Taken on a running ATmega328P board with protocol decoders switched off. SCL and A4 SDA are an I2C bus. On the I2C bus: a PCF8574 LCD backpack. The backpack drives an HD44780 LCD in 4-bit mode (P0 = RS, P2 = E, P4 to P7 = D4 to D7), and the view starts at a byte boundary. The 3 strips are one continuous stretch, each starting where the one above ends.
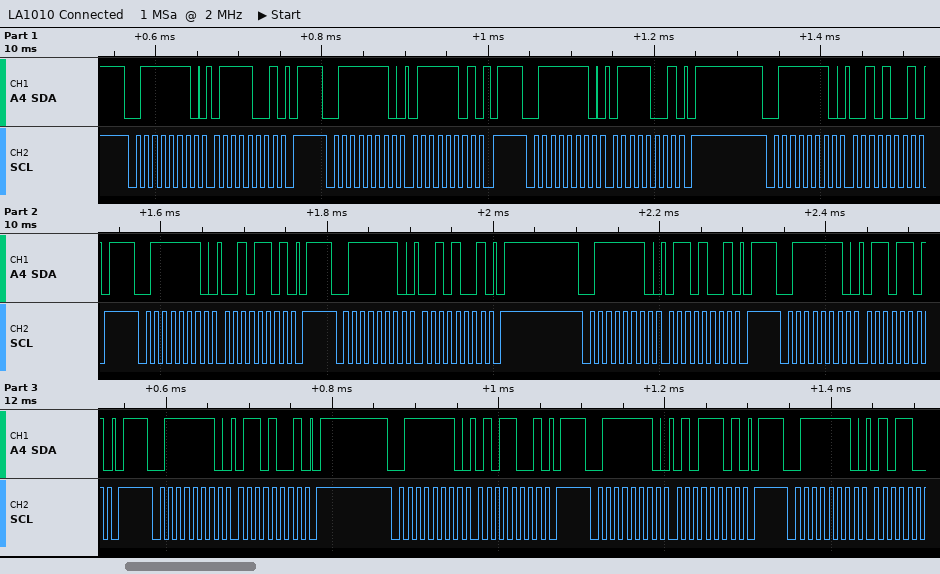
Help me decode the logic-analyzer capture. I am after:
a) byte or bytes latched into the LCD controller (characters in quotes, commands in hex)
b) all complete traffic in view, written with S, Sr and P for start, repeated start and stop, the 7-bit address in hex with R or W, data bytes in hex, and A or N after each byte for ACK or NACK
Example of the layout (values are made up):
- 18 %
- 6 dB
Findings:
- 'r'
- S 3FW A 79 A P S 3FW A 7D A P S 3FW A 79 A P S 3FW A 29 A P S 3FW A 2D A P S 3FW A 29 A P S 3FW A 69 A P S 3FW A 6D A P S 3FW A 69 A P S 3FW A 59 A P S 3FW A 5D A P S 3FW A
